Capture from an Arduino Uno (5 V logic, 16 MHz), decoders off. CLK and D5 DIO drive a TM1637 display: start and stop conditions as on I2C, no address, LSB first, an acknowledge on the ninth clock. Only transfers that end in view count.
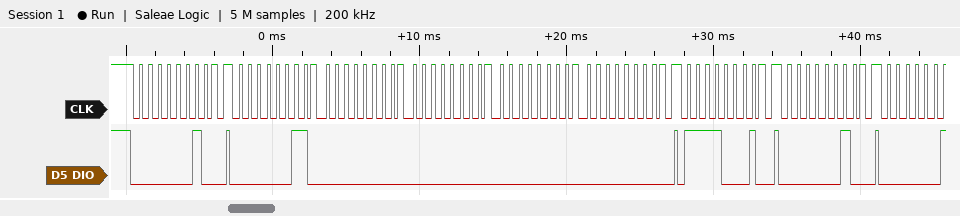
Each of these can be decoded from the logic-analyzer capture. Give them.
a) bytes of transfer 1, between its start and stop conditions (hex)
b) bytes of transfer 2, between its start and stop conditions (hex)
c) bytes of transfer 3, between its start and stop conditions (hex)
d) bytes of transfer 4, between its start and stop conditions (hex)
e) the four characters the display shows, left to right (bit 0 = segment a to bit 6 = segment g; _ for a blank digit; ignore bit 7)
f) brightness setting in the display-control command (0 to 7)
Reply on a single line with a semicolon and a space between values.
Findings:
40; C0 00 00 00 00; 8F; 40; ____; 7
